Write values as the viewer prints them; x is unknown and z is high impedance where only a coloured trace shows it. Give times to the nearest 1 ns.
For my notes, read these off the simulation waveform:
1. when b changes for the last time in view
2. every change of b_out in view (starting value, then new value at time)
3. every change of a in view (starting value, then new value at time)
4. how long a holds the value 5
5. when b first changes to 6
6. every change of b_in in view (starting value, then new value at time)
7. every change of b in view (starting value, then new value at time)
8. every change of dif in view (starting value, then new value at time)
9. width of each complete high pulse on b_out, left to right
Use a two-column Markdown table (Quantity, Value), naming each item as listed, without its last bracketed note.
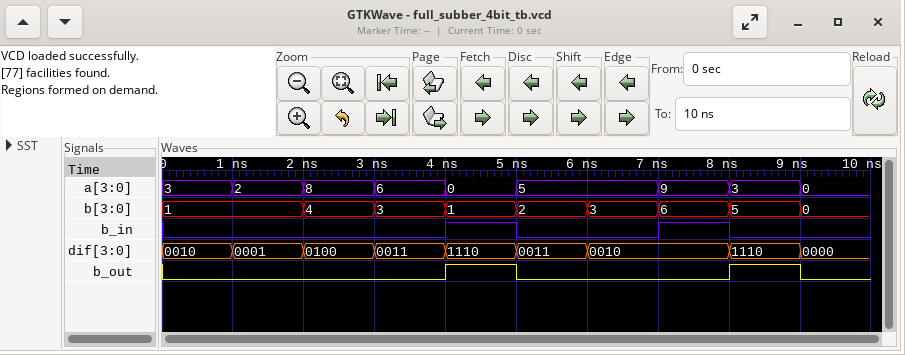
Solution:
| Quantity | Value |
|---|---|
| when b changes for the last time in view | 9 ns |
| every change of b_out in view | 0, 1 at 4 ns, 0 at 5 ns, 1 at 8 ns, 0 at 9 ns |
| every change of a in view | 3, 2 at 1 ns, 8 at 2 ns, 6 at 3 ns, 0 at 4 ns, 5 at 5 ns, 9 at 7 ns, 3 at 8 ns, 0 at 9 ns |
| how long a holds the value 5 | 2 ns |
| when b first changes to 6 | 7 ns |
| every change of b_in in view | 0, 1 at 4 ns, 0 at 5 ns, 1 at 7 ns, 0 at 8 ns |
| every change of b in view | 1, 4 at 2 ns, 3 at 3 ns, 1 at 4 ns, 2 at 5 ns, 3 at 6 ns, 6 at 7 ns, 5 at 8 ns, 0 at 9 ns |
| every change of dif in view | 0010, 0001 at 1 ns, 0100 at 2 ns, 0011 at 3 ns, 1110 at 4 ns, 0011 at 5 ns, 0010 at 6 ns, 1110 at 8 ns, 0000 at 9 ns |
| width of each complete high pulse on b_out, left to right | 1 ns, 1 ns |
